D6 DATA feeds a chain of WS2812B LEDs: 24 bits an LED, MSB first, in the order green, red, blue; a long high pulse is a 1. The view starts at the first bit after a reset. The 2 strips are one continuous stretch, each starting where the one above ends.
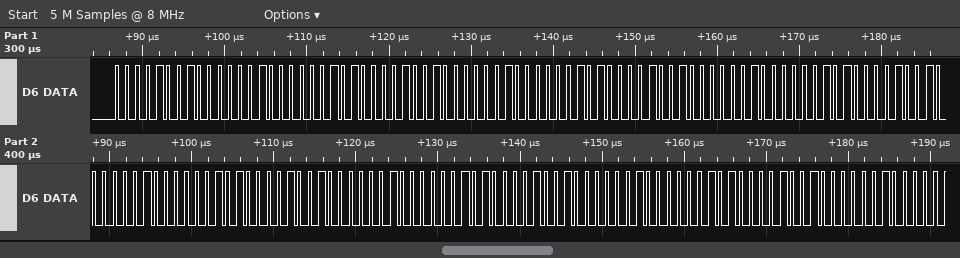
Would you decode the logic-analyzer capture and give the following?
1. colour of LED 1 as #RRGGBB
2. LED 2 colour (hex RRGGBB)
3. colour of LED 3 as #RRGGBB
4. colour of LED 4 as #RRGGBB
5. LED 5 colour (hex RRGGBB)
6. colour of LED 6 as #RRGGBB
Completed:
#020905
#020905
#020905
#020905
#020905
#020905
